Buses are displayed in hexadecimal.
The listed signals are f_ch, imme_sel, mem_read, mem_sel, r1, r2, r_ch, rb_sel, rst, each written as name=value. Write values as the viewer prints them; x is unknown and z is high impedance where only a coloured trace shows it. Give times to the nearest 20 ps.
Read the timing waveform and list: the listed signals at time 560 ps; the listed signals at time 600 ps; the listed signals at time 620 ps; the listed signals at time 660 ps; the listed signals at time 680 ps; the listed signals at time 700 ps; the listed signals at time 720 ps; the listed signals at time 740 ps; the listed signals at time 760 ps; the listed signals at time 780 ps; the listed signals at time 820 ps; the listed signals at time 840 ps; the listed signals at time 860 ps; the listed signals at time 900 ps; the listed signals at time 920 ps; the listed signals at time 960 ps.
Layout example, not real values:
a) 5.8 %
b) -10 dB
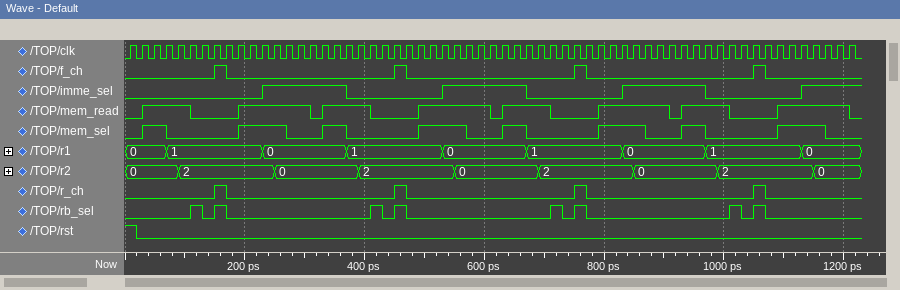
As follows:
a) f_ch=0, imme_sel=1, mem_read=1, mem_sel=1, r1=0, r2=0, r_ch=0, rb_sel=0, rst=0
b) f_ch=0, imme_sel=1, mem_read=1, mem_sel=0, r1=0, r2=0, r_ch=0, rb_sel=0, rst=0
c) f_ch=0, imme_sel=1, mem_read=0, mem_sel=0, r1=0, r2=0, r_ch=0, rb_sel=0, rst=0
d) f_ch=0, imme_sel=1, mem_read=1, mem_sel=1, r1=0, r2=0, r_ch=0, rb_sel=0, rst=0
e) f_ch=0, imme_sel=0, mem_read=1, mem_sel=0, r1=1, r2=0, r_ch=0, rb_sel=0, rst=0
f) f_ch=0, imme_sel=0, mem_read=1, mem_sel=0, r1=1, r2=2, r_ch=0, rb_sel=0, rst=0
g) f_ch=0, imme_sel=0, mem_read=0, mem_sel=0, r1=1, r2=2, r_ch=0, rb_sel=1, rst=0
h) f_ch=0, imme_sel=0, mem_read=0, mem_sel=0, r1=1, r2=2, r_ch=0, rb_sel=0, rst=0
i) f_ch=1, imme_sel=0, mem_read=0, mem_sel=0, r1=1, r2=2, r_ch=1, rb_sel=1, rst=0
j) f_ch=0, imme_sel=0, mem_read=0, mem_sel=0, r1=1, r2=2, r_ch=0, rb_sel=0, rst=0
k) f_ch=0, imme_sel=0, mem_read=1, mem_sel=1, r1=1, r2=2, r_ch=0, rb_sel=0, rst=0
l) f_ch=0, imme_sel=1, mem_read=1, mem_sel=1, r1=0, r2=2, r_ch=0, rb_sel=0, rst=0
m) f_ch=0, imme_sel=1, mem_read=1, mem_sel=1, r1=0, r2=0, r_ch=0, rb_sel=0, rst=0
n) f_ch=0, imme_sel=1, mem_read=1, mem_sel=0, r1=0, r2=0, r_ch=0, rb_sel=0, rst=0
o) f_ch=0, imme_sel=1, mem_read=0, mem_sel=0, r1=0, r2=0, r_ch=0, rb_sel=0, rst=0
p) f_ch=0, imme_sel=1, mem_read=1, mem_sel=1, r1=0, r2=0, r_ch=0, rb_sel=0, rst=0
